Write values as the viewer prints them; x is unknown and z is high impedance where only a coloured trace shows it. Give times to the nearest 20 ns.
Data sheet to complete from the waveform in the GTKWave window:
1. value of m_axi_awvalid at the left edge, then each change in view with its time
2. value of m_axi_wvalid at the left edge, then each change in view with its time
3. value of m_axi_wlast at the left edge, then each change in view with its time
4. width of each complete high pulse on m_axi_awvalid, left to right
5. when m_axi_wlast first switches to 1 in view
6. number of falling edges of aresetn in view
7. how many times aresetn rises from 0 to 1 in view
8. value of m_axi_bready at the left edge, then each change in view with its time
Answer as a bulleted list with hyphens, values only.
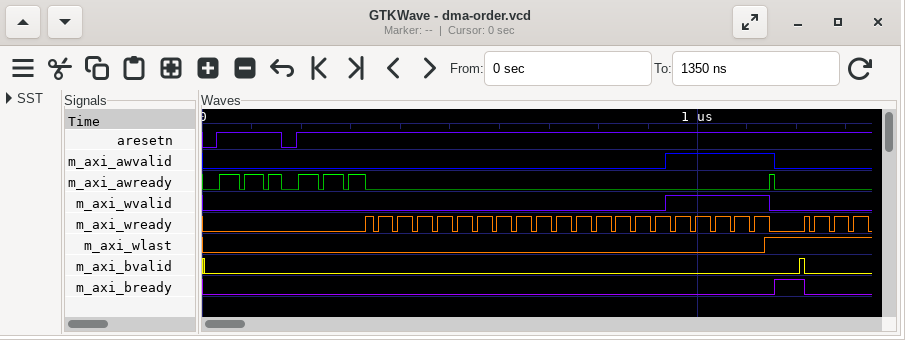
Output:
- 0, 1 at 940 ns, 0 at 1160 ns
- 0, 1 at 940 ns, 0 at 1140 ns
- 0, 1 at 1140 ns
- 220 ns
- 1140 ns
- 1
- 2
- 0, 1 at 1160 ns, 0 at 1220 ns
